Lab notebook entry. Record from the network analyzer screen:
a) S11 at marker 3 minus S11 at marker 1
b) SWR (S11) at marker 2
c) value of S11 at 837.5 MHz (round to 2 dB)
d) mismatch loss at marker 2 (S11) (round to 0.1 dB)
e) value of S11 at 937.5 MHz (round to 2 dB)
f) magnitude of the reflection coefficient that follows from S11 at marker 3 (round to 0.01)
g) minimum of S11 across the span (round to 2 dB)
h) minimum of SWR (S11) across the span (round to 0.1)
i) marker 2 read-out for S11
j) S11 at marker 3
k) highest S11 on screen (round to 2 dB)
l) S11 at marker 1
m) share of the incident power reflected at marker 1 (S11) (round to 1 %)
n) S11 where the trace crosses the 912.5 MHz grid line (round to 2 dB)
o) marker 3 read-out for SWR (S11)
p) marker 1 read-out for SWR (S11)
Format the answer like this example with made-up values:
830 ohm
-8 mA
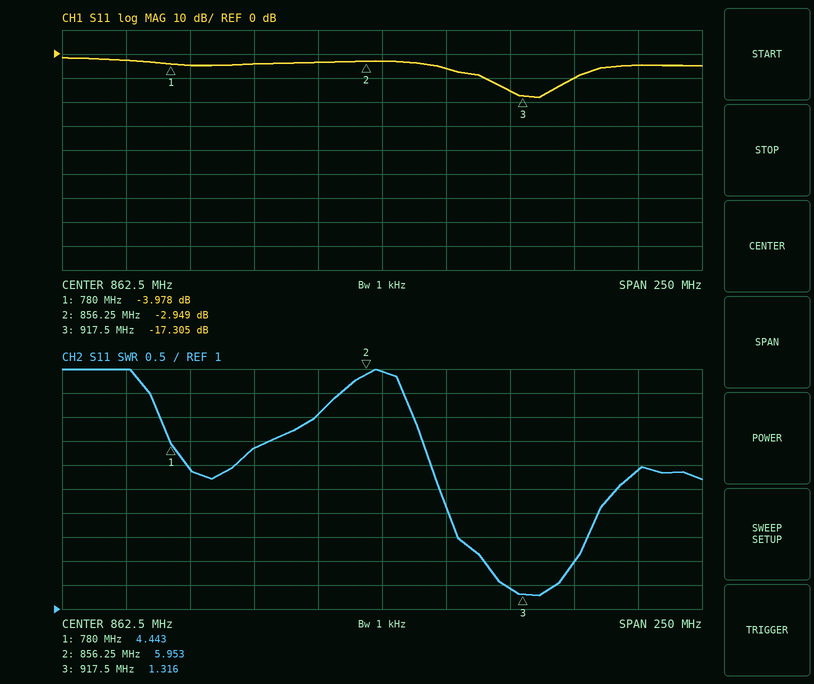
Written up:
-13.327 dB
5.953
-4 dB
3.1 dB
-10 dB
0.14
-18 dB
1.3
-2.949 dB
-17.305 dB
-2 dB
-3.978 dB
40 %
-16 dB
1.316
4.443
